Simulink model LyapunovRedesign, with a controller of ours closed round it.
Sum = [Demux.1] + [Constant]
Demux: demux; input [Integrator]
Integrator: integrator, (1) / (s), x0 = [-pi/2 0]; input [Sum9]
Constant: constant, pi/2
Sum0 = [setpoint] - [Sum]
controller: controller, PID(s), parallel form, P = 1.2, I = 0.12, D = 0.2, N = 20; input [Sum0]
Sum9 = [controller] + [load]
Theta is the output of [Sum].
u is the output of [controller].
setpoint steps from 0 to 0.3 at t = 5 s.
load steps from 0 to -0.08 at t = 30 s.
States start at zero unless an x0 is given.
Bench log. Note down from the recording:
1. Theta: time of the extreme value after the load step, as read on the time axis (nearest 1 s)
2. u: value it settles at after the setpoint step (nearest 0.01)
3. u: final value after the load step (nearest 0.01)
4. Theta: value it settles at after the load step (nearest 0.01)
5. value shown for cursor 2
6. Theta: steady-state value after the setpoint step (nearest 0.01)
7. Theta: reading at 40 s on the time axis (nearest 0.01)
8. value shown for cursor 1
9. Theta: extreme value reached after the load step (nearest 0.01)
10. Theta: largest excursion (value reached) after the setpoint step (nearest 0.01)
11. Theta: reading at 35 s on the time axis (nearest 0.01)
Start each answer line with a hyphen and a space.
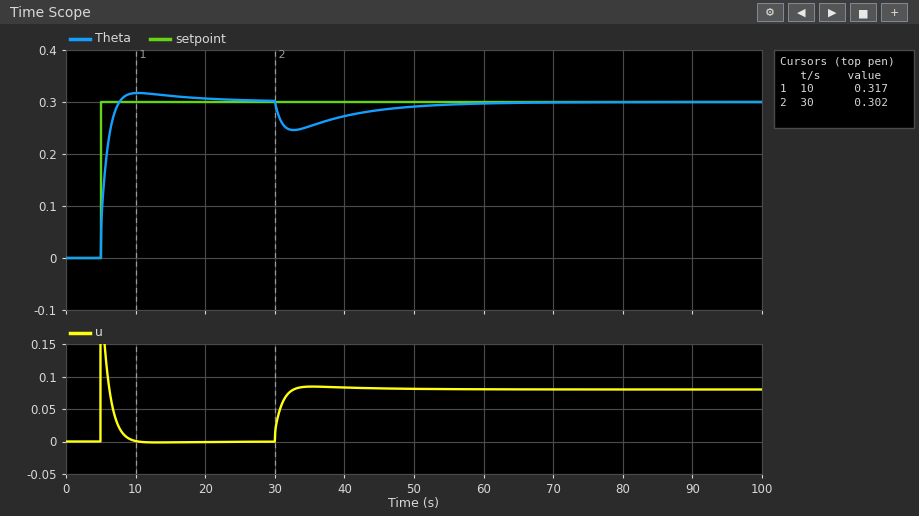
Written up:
- 33 s
- 0.00
- 0.08
- 0.30
- 0.302
- 0.30
- 0.27
- 0.317
- 0.25
- 0.32
- 0.25
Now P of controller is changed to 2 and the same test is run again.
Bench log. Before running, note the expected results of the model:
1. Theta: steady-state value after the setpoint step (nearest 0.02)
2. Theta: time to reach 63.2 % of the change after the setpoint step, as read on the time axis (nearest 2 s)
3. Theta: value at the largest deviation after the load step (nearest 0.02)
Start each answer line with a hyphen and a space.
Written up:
- 0.30
- 6 s
- 0.26
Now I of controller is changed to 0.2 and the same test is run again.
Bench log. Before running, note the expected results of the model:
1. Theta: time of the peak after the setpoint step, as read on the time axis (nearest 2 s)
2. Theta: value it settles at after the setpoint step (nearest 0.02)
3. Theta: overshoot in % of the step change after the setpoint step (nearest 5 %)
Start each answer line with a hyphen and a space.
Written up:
- 10 s
- 0.30
- 10 %
